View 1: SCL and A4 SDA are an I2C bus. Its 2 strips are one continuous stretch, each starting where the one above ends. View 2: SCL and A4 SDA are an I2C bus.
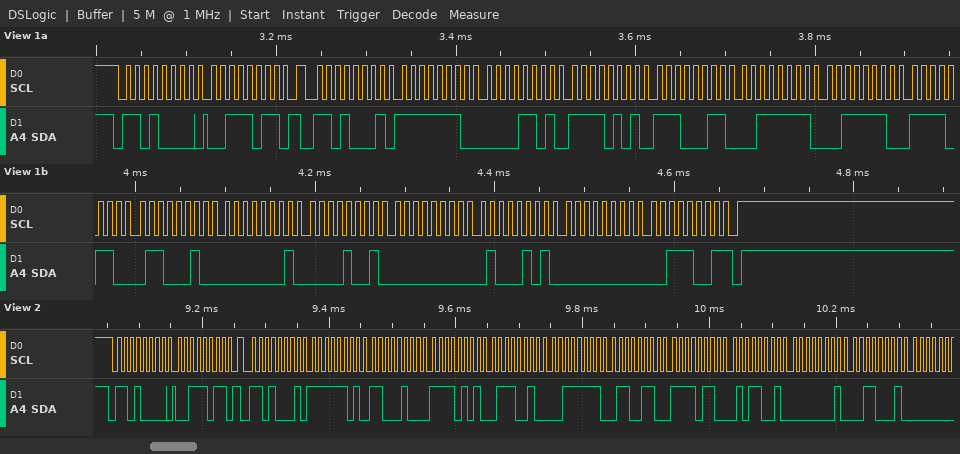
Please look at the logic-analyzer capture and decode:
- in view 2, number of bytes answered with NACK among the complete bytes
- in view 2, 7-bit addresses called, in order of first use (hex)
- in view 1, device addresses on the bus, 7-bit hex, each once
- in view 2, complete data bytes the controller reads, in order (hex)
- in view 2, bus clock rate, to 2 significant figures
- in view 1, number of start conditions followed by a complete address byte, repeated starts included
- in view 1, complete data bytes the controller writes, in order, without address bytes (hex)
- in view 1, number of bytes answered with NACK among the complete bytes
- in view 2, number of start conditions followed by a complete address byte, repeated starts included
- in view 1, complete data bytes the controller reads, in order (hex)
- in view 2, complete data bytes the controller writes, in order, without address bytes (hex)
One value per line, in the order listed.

0
0x68
0x68
FD C4 F5 72 3F 66 F6 59 01 31
100 kHz
2
3B
1
2
FE 0D F5 E3 3F 3E F6 62 01 09 00 45 00 39
3B
